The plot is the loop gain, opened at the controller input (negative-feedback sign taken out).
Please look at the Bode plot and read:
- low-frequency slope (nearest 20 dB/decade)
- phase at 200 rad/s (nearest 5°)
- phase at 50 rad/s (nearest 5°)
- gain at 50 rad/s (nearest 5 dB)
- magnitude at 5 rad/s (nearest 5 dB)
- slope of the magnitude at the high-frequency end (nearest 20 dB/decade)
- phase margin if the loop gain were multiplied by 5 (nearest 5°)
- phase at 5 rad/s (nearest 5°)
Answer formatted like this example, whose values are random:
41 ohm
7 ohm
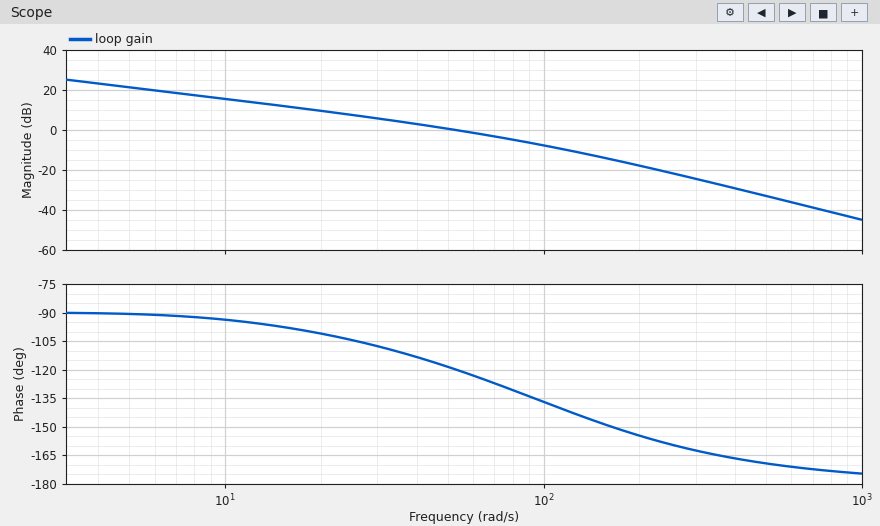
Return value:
-20 dB/decade
-155°
-120°
0 dB
20 dB
-40 dB/decade
30°
-90°
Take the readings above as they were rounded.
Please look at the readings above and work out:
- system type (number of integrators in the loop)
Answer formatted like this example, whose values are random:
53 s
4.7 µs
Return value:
1
